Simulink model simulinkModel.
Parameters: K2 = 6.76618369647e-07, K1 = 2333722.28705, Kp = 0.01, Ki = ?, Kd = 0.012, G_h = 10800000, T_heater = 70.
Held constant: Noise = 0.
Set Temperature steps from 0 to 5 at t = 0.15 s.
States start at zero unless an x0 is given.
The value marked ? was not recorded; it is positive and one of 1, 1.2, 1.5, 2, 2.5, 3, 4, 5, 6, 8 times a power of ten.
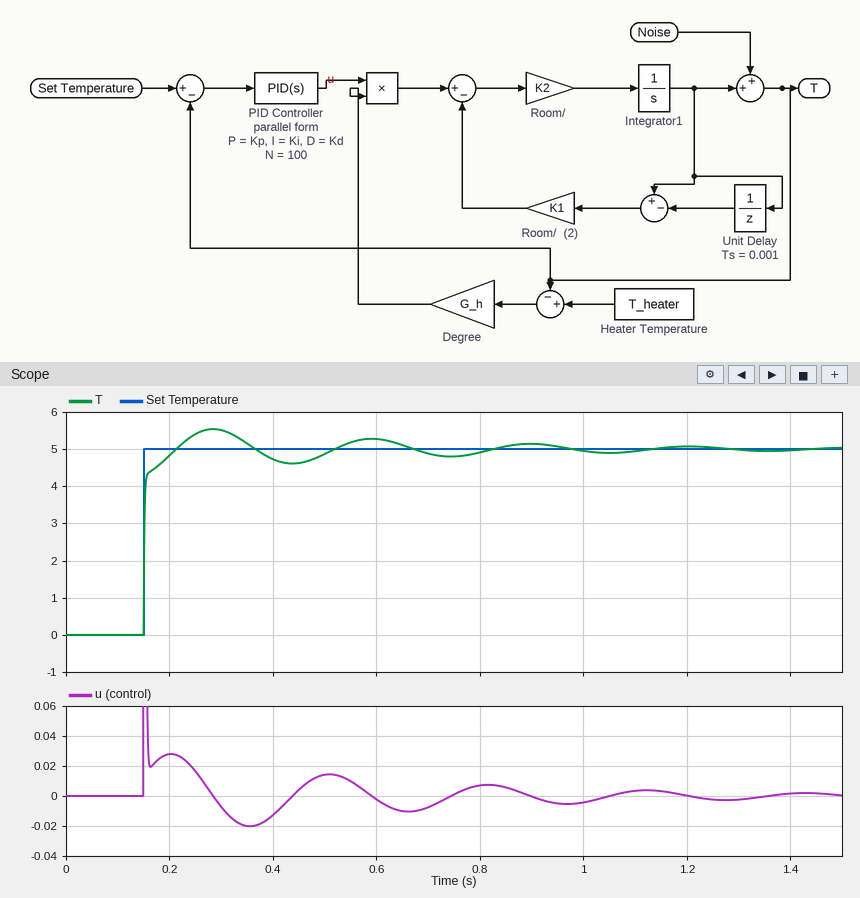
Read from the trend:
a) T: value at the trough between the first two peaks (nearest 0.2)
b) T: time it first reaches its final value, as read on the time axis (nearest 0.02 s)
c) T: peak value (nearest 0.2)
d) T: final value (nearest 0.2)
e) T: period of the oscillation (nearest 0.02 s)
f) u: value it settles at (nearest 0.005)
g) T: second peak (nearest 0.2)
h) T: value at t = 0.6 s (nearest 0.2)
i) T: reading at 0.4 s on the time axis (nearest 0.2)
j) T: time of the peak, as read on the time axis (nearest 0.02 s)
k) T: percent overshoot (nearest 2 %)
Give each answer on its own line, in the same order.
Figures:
4.6
0.22 s
5.6
5.0
0.30 s
0.000
5.2
5.2
4.8
0.28 s
10 %
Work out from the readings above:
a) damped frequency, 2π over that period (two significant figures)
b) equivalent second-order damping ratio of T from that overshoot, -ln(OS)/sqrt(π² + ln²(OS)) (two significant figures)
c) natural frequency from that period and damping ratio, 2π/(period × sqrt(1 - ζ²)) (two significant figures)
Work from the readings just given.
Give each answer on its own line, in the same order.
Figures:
21 rad/s
0.59
26 rad/s
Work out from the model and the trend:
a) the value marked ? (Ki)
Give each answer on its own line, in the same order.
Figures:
6
